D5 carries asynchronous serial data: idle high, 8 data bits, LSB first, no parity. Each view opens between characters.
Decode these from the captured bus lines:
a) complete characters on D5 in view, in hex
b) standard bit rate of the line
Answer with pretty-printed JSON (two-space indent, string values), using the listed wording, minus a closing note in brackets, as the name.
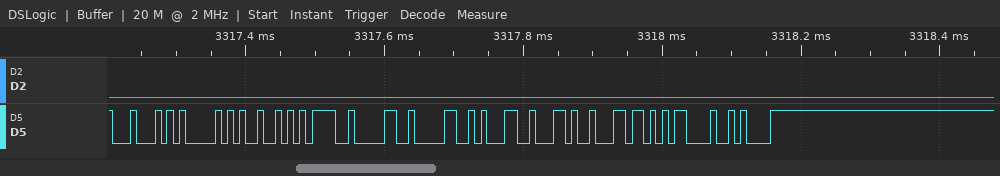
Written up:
{
  "complete characters on D5 in view, in hex": "44, 41, 49, 3D, 30, 30, 31, 2C, 6C, 0D, 0A",
  "standard bit rate of the line": "115200 baud"
}
